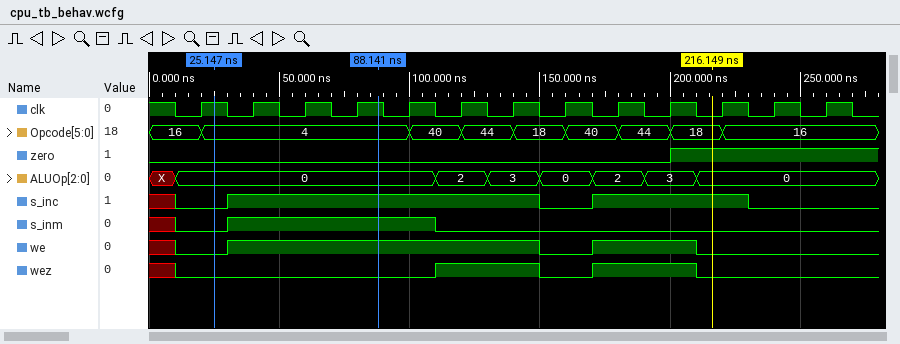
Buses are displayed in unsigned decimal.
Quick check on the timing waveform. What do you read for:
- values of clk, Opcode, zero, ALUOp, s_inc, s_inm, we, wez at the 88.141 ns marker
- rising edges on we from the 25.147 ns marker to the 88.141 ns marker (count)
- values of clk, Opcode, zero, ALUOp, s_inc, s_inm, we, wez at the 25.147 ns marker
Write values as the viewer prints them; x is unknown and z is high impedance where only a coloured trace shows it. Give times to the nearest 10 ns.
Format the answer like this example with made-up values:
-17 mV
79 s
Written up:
clk=1, Opcode=4, zero=0, ALUOp=0, s_inc=1, s_inm=1, we=1, wez=0
1
clk=1, Opcode=4, zero=0, ALUOp=0, s_inc=0, s_inm=0, we=0, wez=0
